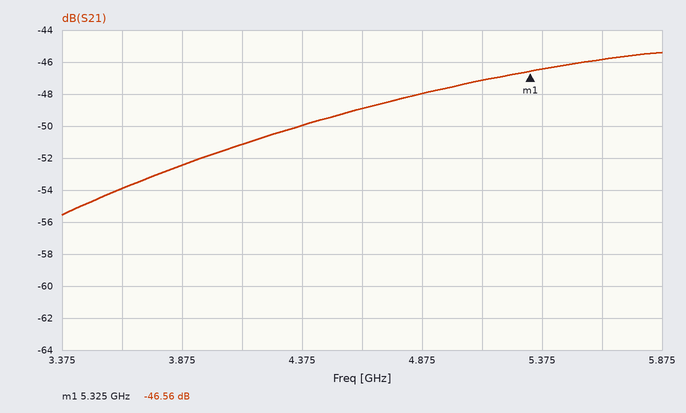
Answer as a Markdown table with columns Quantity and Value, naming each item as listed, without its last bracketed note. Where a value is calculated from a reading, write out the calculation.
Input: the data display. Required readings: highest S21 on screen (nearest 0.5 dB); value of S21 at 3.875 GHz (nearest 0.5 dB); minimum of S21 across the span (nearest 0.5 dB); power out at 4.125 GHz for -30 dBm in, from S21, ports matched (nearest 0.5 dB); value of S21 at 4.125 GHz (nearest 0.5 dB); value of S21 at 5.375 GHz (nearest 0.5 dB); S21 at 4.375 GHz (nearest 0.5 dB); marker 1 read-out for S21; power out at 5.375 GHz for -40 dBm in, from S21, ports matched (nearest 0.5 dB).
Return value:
| Quantity | Value |
|---|---|
| highest S21 on screen | -45.5 dB |
| value of S21 at 3.875 GHz | -52.5 dB |
| minimum of S21 across the span | -55.5 dB |
| power out at 4.125 GHz for -30 dBm in, from S21, ports matched | -30 dBm + (-51.0 dB) = -81.0 dBm |
| value of S21 at 4.125 GHz | -51.0 dB |
| value of S21 at 5.375 GHz | -46.5 dB |
| S21 at 4.375 GHz | -50.0 dB |
| marker 1 read-out for S21 | -46.56 dB |
| power out at 5.375 GHz for -40 dBm in, from S21, ports matched | -40 dBm + (-46.5 dB) = -86.5 dBm |
